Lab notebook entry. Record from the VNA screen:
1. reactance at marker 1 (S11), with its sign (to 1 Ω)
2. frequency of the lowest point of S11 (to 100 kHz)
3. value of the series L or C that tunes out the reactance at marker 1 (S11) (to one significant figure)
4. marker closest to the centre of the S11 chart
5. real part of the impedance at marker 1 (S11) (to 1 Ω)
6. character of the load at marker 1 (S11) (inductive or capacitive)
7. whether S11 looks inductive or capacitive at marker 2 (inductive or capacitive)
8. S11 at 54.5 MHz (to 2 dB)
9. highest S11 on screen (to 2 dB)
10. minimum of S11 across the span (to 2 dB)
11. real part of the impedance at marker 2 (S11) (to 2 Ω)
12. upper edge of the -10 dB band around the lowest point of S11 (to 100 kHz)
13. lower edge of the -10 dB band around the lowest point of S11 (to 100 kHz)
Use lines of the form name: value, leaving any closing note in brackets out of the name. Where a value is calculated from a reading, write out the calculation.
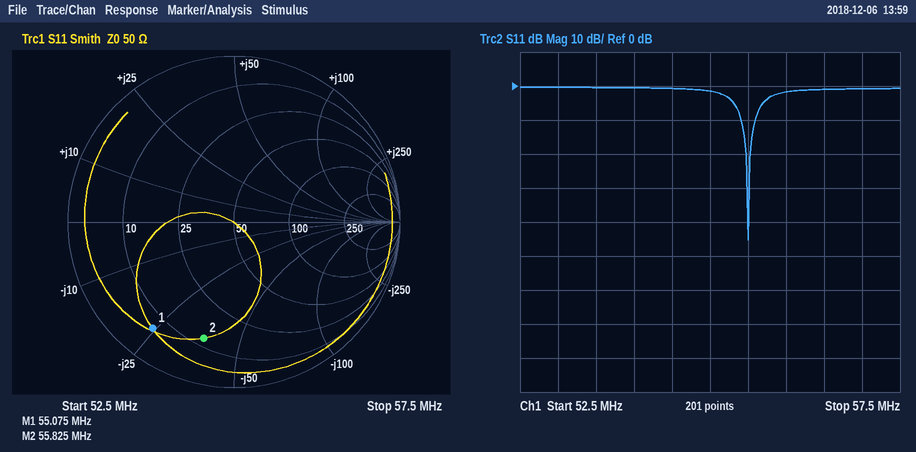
reactance at marker 1 (S11), with its sign: -24 Ω
frequency of the lowest point of S11: 55.5 MHz
value of the series L or C that tunes out the reactance at marker 1 (S11): L = 24 Ω/(2π × 55.075 MHz) ≈ 69.4 nH, so 70 nH to one significant figure
marker closest to the centre of the S11 chart: marker 2
real part of the impedance at marker 1 (S11): 7 Ω
character of the load at marker 1 (S11): capacitive
whether S11 looks inductive or capacitive at marker 2: capacitive
S11 at 54.5 MHz: 0 dB
highest S11 on screen: 0 dB
minimum of S11 across the span: -46 dB
real part of the impedance at marker 2 (S11): 12 Ω
upper edge of the -10 dB band around the lowest point of S11: 55.6 MHz
lower edge of the -10 dB band around the lowest point of S11: 55.4 MHz
